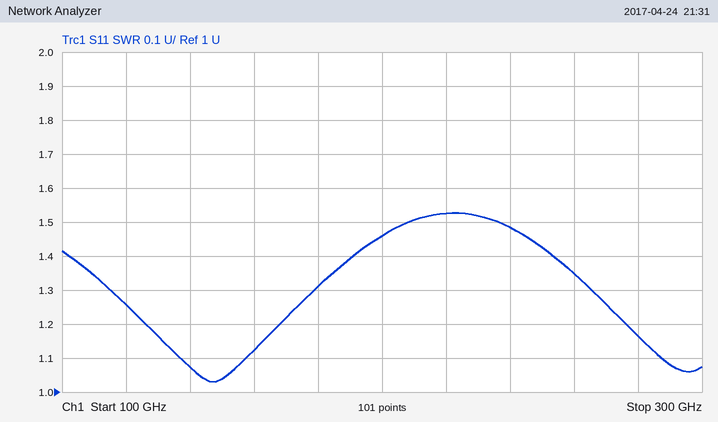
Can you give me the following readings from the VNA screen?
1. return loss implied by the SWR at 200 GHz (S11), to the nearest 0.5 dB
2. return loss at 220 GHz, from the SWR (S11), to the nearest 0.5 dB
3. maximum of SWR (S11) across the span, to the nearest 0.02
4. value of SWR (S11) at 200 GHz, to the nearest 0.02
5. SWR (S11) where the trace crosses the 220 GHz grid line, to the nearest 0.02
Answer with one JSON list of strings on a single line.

["14.5 dB", "13.5 dB", "1.52", "1.46", "1.52"]
